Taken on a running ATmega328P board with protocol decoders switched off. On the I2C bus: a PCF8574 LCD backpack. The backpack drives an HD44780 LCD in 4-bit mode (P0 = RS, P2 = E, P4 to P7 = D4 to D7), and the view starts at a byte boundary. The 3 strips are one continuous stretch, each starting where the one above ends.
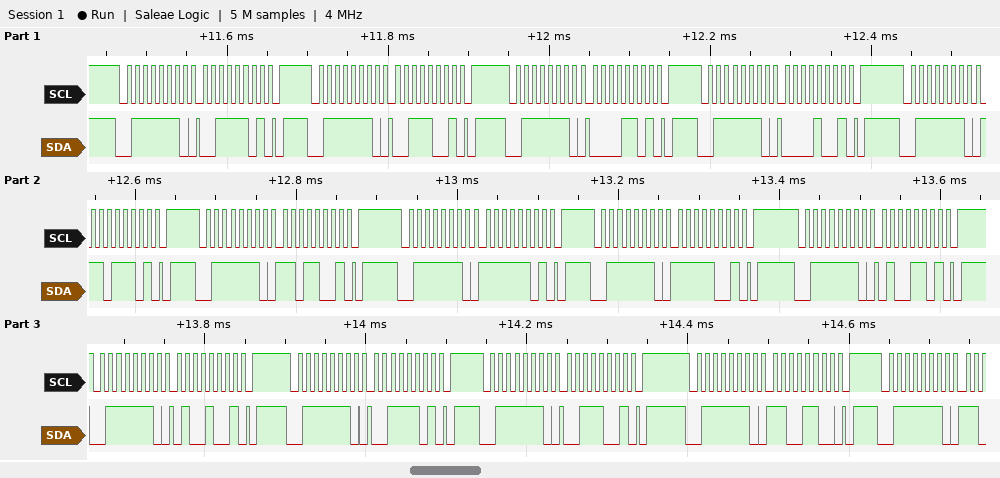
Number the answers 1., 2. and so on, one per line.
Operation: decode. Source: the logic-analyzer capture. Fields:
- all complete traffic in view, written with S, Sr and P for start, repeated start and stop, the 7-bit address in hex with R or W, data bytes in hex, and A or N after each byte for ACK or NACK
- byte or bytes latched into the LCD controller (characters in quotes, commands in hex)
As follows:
1. S 3FW A 3D A P S 3FW A 39 A P S 3FW A 0D A P S 3FW A 09 A P S 3FW A DD A P S 3FW A D9 A P S 3FW A FD A P S 3FW A F9 A P S 3FW A 4D A P S 3FW A 49 A P S 3FW A 3D A P S 3FW A 39 A P S 3FW A CC A P S 3FW A
2. '0' data 0xDF 'C'
